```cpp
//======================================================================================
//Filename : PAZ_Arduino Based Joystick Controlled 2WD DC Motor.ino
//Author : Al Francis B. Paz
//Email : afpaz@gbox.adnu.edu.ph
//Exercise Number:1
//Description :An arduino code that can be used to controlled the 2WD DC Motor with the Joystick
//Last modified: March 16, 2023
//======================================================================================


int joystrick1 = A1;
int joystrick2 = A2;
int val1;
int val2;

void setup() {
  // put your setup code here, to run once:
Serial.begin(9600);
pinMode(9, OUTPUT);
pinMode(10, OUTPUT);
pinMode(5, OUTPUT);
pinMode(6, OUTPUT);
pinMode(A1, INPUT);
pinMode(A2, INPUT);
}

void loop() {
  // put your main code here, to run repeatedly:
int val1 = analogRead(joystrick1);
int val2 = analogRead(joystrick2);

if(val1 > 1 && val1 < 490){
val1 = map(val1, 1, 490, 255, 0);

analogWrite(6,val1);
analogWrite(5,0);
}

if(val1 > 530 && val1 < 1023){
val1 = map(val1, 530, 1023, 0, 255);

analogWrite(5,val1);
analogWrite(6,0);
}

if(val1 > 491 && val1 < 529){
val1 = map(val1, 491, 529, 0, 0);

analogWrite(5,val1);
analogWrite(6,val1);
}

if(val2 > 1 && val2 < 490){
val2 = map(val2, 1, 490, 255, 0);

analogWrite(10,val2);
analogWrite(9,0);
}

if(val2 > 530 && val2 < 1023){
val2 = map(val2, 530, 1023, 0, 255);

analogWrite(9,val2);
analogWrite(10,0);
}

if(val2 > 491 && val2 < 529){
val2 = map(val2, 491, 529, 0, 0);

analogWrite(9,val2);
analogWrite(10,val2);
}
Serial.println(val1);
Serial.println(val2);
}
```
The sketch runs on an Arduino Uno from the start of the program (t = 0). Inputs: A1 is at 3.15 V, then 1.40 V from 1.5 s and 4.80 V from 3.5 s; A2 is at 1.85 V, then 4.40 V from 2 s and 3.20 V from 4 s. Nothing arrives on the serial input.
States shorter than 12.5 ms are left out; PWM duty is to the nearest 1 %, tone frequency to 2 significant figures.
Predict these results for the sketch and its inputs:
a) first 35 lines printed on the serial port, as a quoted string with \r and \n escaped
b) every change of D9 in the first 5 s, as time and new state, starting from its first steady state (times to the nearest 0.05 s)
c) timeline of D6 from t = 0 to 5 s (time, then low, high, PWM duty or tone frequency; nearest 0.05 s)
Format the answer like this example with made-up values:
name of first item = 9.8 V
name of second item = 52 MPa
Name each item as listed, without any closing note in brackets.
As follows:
first 35 lines printed on the serial port, as a quoted string with \r and \n escaped = "59\r\n59\r\n59\r\n59\r\n59\r\n59\r\n59\r\n59\r\n59\r\n59\r\n59\r\n59\r\n59\r\n59\r\n59\r\n59\r\n59\r\n59\r\n59\r\n59\r\n59\r\n59\r\n59\r\n59\r\n59\r\n59\r\n59\r\n59\r\n59\r\n59\r\n59\r\n59\r\n59\r\n59\r\n59\r\n"
every change of D9 in the first 5 s, as time and new state, starting from its first steady state = 0 s low; 2 s PWM 75 %; 4 s PWM 25 %
timeline of D6 from t = 0 to 5 s = 0 s low; 1.5 s PWM 42 %; 3.5 s low
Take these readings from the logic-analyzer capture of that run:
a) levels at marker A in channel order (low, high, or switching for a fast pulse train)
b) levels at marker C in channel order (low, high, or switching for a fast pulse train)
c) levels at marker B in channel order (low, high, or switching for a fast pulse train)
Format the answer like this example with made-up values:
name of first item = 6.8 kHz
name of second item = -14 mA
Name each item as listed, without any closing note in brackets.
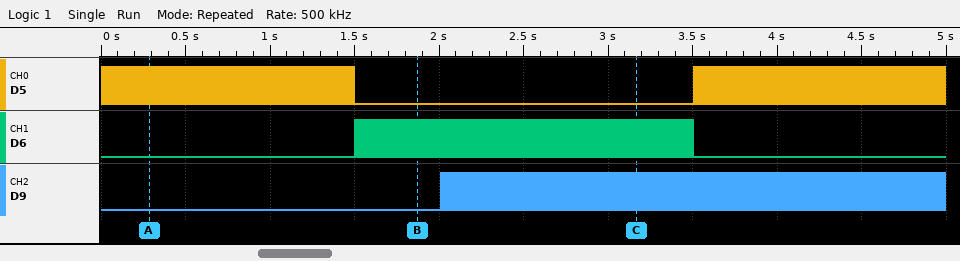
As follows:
levels at marker A in channel order = D5 switching, D6 low, D9 low
levels at marker C in channel order = D5 low, D6 switching, D9 switching
levels at marker B in channel order = D5 low, D6 switching, D9 low
